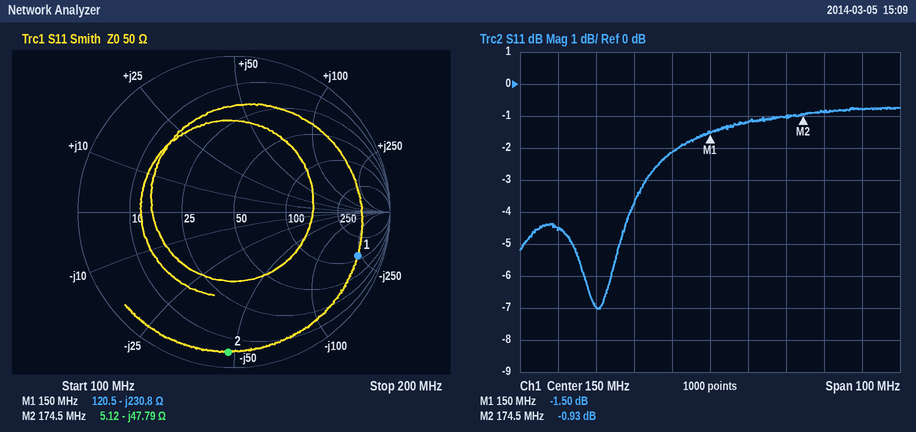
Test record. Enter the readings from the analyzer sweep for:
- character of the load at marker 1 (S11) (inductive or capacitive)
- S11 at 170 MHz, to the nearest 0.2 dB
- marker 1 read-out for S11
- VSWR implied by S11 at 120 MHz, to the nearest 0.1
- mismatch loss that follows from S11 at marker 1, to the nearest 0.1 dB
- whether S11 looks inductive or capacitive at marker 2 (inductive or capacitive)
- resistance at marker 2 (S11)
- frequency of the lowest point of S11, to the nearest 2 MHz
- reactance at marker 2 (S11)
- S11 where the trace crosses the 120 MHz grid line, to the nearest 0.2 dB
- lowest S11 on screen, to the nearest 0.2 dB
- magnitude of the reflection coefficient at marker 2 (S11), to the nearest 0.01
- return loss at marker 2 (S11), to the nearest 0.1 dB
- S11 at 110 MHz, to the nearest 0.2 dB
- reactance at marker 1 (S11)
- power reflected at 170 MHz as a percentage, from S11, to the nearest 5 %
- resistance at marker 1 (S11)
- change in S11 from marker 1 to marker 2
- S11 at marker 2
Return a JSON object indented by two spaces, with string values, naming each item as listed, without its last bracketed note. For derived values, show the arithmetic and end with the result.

{
  "character of the load at marker 1 (S11)": "capacitive",
  "S11 at 170 MHz, to the nearest 0.2 dB": "-1.0 dB",
  "marker 1 read-out for S11": "-1.50 dB",
  "VSWR implied by S11 at 120 MHz, to the nearest 0.1": "|Γ| = 10^(-7/20) = 0.4467; VSWR = (1 + 0.4467)/(1 − 0.4467) ≈ 2.6",
  "mismatch loss that follows from S11 at marker 1, to the nearest 0.1 dB": "−10 log10(1 − 10^(-1.5/10)) ≈ 5.3 dB",
  "whether S11 looks inductive or capacitive at marker 2": "capacitive",
  "resistance at marker 2": "5.12 Ω",
  "frequency of the lowest point of S11, to the nearest 2 MHz": "120 MHz",
  "reactance at marker 2": "-47.79 Ω",
  "S11 where the trace crosses the 120 MHz grid line, to the nearest 0.2 dB": "-7.0 dB",
  "lowest S11 on screen, to the nearest 0.2 dB": "-7.0 dB",
  "magnitude of the reflection coefficient at marker 2 (S11), to the nearest 0.01": "10^(-0.93/20) ≈ 0.90",
  "return loss at marker 2 (S11), to the nearest 0.1 dB": "0.9 dB",
  "S11 at 110 MHz, to the nearest 0.2 dB": "-4.6 dB",
  "reactance at marker 1": "-230.8 Ω",
  "power reflected at 170 MHz as a percentage, from S11, to the nearest 5 %": "10^(-1/10) ≈ 79.4 %, so 80 % to the nearest 5 %",
  "resistance at marker 1": "120.5 Ω",
  "change in S11 from marker 1 to marker 2": "-0.93 − (-1.5) = 0.57 dB",
  "S11 at marker 2": "-0.93 dB"
}
